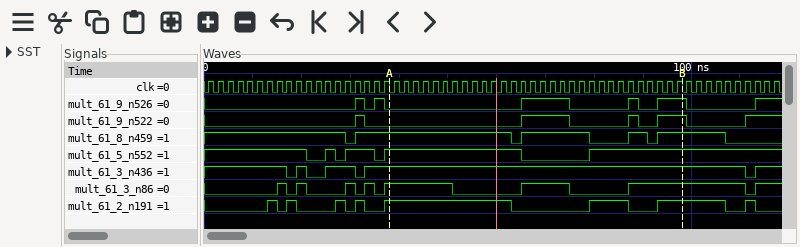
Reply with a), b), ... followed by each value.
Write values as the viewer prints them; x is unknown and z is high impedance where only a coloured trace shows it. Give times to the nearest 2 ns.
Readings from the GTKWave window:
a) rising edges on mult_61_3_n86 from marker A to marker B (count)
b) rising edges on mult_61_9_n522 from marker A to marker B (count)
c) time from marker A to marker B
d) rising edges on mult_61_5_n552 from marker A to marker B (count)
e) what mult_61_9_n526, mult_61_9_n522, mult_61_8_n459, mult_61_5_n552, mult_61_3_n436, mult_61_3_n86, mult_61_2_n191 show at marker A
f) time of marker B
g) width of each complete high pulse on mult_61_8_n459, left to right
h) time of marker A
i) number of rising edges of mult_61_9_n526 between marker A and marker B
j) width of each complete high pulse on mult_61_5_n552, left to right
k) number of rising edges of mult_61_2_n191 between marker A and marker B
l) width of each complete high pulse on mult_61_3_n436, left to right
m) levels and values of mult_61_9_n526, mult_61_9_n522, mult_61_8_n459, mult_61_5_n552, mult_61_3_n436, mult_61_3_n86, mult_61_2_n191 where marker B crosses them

a) 2
b) 3
c) 60 ns
d) 1
e) mult_61_9_n526=0, mult_61_9_n522=0, mult_61_8_n459=1, mult_61_5_n552=1, mult_61_3_n436=1, mult_61_3_n86=1, mult_61_2_n191=1
f) 98 ns
g) 32 ns, 14 ns, 4 ns, 14 ns
h) 38 ns
i) 3
j) 2 ns, 6 ns, 28 ns
k) 2
l) 2 ns, 6 ns, 78 ns
m) mult_61_9_n526=1, mult_61_9_n522=1, mult_61_8_n459=1, mult_61_5_n552=1, mult_61_3_n436=1, mult_61_3_n86=1, mult_61_2_n191=1
